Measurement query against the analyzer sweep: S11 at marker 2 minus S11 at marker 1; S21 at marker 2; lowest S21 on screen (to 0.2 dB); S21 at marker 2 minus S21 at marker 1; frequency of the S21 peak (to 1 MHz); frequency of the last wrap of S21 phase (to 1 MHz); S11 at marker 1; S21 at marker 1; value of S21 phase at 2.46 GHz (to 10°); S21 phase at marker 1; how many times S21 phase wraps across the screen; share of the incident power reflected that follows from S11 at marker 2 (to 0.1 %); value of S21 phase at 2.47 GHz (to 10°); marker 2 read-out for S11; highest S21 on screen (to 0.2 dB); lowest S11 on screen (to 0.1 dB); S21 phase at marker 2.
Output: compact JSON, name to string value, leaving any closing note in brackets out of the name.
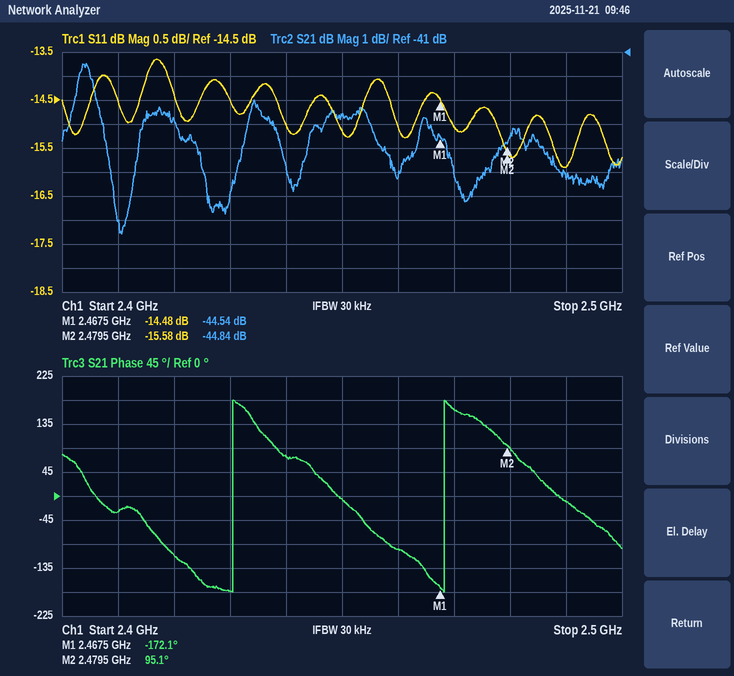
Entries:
{"S11 at marker 2 minus S11 at marker 1": "-1.10 dB", "S21 at marker 2": "-44.84 dB", "lowest S21 on screen": "-48.6 dB", "S21 at marker 2 minus S21 at marker 1": "-0.30 dB", "frequency of the S21 peak": "2.404 GHz", "frequency of the last wrap of S21 phase": "2.468 GHz", "S11 at marker 1": "-14.48 dB", "S21 at marker 1": "-44.54 dB", "value of S21 phase at 2.46 GHz": "-100°", "S21 phase at marker 1": "-172.1°", "how many times S21 phase wraps across the screen": "2", "share of the incident power reflected that follows from S11 at marker 2": "2.8 %", "value of S21 phase at 2.47 GHz": "160°", "marker 2 read-out for S11": "-15.58 dB", "highest S21 on screen": "-41.4 dB", "lowest S11 on screen": "-15.9 dB", "S21 phase at marker 2": "95.1°"}
